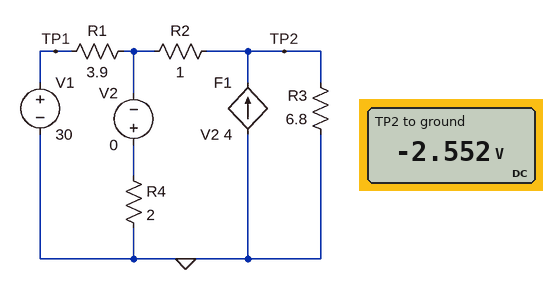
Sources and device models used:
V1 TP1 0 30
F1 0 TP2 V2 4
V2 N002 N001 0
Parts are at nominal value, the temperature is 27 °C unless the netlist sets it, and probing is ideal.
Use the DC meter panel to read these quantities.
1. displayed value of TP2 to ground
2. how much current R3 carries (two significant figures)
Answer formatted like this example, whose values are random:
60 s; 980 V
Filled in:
-2.552 V; 380 mA
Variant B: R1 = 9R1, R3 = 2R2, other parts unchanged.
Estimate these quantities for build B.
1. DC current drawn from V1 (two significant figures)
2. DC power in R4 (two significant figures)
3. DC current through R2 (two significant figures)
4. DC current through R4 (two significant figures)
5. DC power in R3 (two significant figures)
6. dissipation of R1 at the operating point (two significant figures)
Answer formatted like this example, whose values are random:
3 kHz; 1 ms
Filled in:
3.1 A; 1.0 W; 2.4 A; 720 mA; 440 mW; 90 W
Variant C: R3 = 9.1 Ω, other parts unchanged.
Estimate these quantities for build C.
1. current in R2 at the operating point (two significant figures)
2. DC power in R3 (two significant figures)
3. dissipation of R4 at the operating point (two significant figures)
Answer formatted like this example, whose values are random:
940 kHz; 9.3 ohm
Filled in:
5.5 A; 750 mW; 4.2 W
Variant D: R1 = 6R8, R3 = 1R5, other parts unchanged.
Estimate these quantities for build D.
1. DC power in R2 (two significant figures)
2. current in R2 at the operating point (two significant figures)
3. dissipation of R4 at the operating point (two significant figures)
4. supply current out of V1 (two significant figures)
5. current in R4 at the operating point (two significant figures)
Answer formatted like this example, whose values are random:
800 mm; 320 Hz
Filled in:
9.9 W; 3.1 A; 1.9 W; 4.1 A; 980 mA
